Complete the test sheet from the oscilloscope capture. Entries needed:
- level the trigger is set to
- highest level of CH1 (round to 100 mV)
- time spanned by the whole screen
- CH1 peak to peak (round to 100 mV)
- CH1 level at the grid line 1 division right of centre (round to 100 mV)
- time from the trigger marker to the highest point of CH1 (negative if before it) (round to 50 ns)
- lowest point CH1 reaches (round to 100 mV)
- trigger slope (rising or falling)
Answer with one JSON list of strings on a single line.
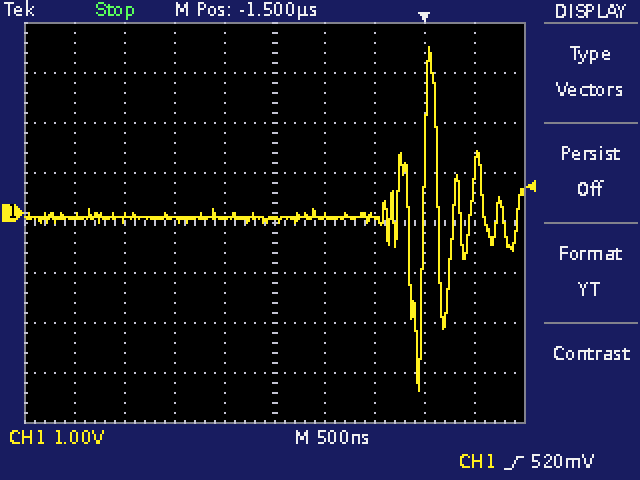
["520 mV", "3.3 V", "5 µs", "6.9 V", "-100 mV", "+50 ns", "-3.6 V", "rising"]
